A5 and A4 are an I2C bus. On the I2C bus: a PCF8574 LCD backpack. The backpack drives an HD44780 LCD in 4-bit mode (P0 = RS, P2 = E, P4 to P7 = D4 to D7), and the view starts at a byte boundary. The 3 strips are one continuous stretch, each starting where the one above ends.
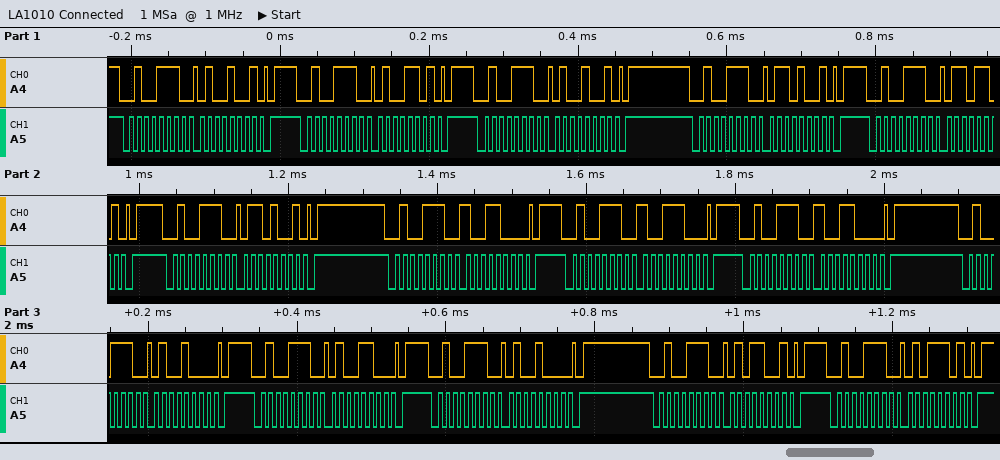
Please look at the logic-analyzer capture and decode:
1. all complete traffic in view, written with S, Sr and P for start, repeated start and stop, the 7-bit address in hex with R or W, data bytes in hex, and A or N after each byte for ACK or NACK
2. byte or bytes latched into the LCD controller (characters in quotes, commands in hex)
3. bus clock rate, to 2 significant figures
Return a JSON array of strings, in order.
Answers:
["S 27W A 49 A P S 27W A 4D A P S 27W A 49 A P S 27W A 69 A P S 27W A 6D A P S 27W A 69 A P S 27W A 98 A P S 27W A 9C A P S 27W A 98 A P S 27W A 48 A P S 27W A 4C A P S 27W A 48 A P S 27W A 59 A P S 27W A 5D A P", "'F' 0x94", "100 kHz"]
